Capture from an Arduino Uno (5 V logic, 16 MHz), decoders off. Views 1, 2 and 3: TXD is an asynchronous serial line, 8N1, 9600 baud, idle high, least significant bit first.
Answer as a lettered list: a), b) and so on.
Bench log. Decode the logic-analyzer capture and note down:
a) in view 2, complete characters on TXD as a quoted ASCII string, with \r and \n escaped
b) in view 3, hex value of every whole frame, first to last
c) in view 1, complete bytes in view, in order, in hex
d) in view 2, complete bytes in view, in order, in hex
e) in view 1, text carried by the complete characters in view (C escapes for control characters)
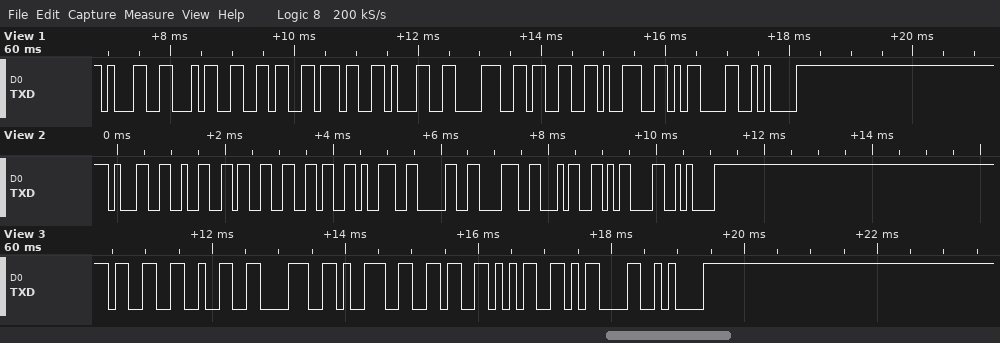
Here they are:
a) "12369084\r\n"
b) 33 32 38 39 36 35 0D 0A
c) 0x31 0x34 0x36 0x37 0x31 0x38 0x33 0x39 0x0D 0x0A
d) 0x31 0x32 0x33 0x36 0x39 0x30 0x38 0x34 0x0D 0x0A
e) "14671839\r\n"
